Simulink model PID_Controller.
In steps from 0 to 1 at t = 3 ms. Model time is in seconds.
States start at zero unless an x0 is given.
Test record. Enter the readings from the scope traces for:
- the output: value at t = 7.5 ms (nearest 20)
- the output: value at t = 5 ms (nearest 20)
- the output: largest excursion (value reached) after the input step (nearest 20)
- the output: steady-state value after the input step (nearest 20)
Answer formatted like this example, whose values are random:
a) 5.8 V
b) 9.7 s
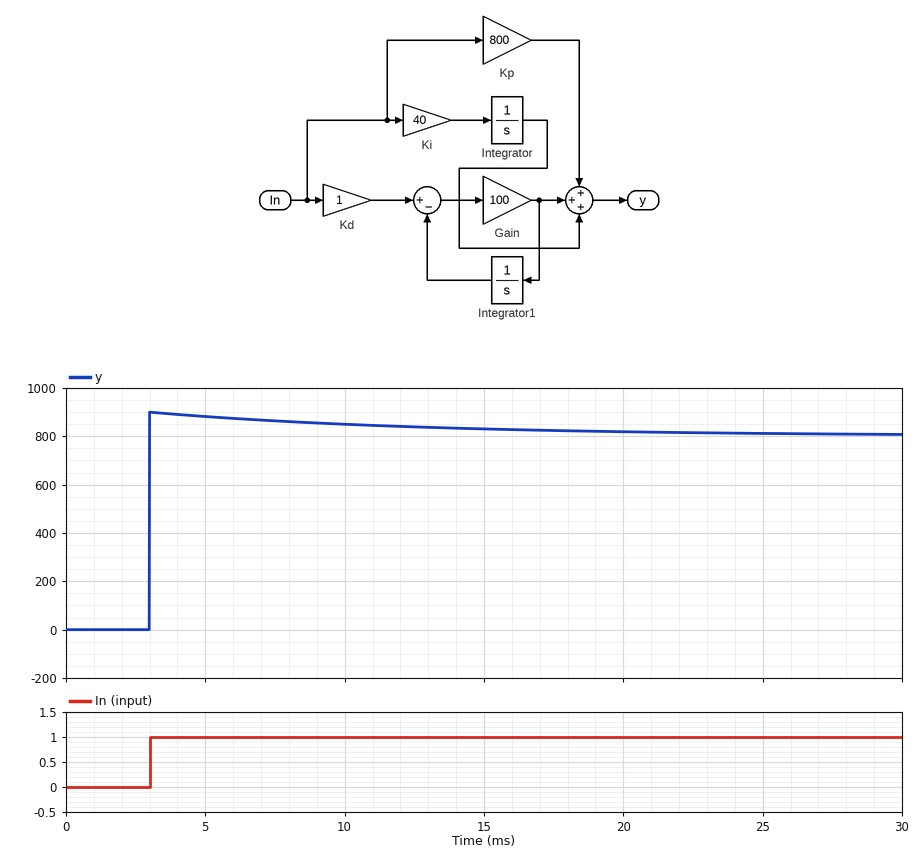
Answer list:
a) 860
b) 880
c) 900
d) 800
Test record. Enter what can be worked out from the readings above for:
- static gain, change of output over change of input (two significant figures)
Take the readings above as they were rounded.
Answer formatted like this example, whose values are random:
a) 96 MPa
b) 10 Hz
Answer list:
a) 800
